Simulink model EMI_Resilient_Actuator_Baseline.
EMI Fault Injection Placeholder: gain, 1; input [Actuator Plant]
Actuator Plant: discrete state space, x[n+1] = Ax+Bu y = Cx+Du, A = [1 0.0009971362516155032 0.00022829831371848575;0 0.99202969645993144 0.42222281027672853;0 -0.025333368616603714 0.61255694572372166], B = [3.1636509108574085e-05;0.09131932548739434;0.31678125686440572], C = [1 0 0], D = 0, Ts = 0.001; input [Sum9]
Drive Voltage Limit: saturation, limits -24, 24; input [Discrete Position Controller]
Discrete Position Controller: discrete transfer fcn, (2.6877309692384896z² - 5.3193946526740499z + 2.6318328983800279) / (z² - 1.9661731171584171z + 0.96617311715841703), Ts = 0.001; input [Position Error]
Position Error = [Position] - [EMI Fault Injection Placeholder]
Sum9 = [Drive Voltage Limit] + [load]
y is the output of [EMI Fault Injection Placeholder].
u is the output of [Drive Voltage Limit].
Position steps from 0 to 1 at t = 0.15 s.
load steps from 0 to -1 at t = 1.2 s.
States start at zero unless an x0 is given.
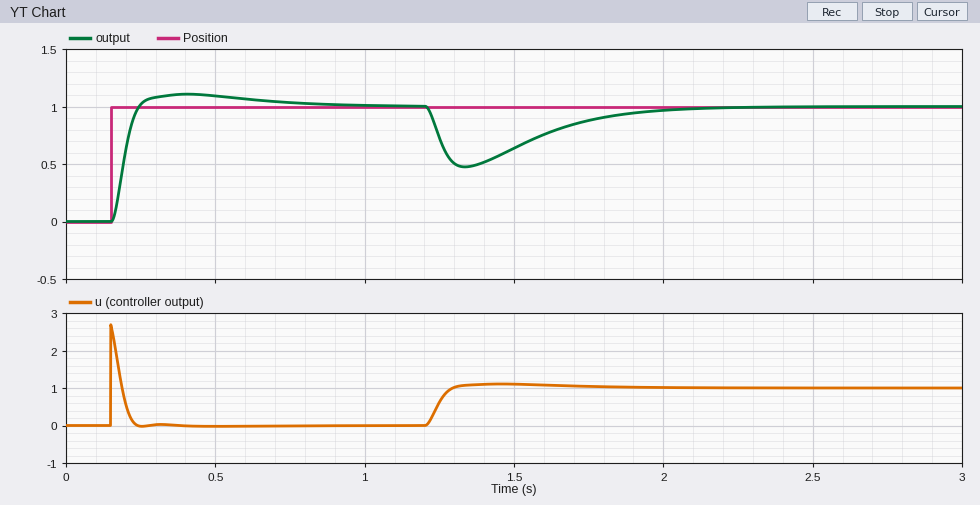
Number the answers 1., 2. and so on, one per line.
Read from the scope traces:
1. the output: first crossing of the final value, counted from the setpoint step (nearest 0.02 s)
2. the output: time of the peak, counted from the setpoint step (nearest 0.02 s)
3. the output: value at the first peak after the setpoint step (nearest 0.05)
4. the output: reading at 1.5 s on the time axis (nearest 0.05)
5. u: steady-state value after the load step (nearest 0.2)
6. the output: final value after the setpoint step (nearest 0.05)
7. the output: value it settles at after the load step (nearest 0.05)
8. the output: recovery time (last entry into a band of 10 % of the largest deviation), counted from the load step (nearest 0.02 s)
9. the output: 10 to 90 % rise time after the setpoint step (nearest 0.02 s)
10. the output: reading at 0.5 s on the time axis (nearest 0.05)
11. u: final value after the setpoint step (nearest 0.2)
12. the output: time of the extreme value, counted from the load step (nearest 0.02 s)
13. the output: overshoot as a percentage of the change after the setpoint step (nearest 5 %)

1. 0.10 s
2. 0.26 s
3. 1.10
4. 0.65
5. 1.0
6. 1.00
7. 1.00
8. 0.72 s
9. 0.06 s
10. 1.10
11. 0.0
12. 0.14 s
13. 10 %
